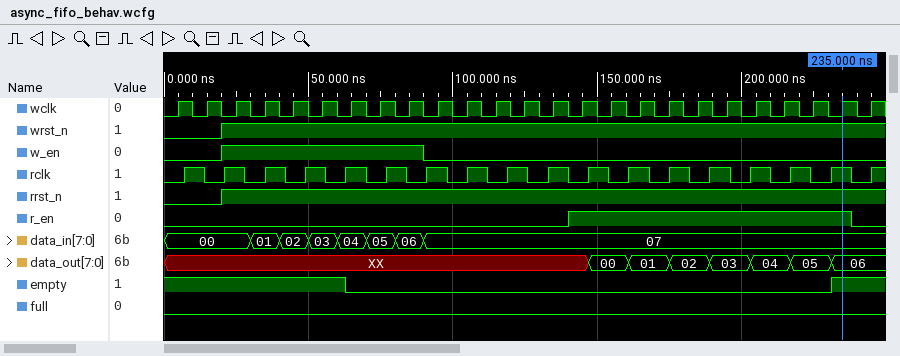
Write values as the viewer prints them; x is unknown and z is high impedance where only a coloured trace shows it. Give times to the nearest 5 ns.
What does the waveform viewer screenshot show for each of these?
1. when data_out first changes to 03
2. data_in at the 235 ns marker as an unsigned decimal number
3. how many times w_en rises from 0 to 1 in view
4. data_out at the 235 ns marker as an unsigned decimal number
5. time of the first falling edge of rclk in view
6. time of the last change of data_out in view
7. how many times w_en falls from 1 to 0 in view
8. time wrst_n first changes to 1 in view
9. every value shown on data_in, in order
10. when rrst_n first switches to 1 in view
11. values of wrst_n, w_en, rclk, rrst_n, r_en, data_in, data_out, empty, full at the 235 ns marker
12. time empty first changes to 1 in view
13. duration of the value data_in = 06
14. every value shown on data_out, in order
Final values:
190 ns
7
1
6
15 ns
230 ns
1
20 ns
00, 01, 02, 03, 04, 05, 06, 07
20 ns
wrst_n=1, w_en=0, rclk=1, rrst_n=1, r_en=1, data_in=07, data_out=06, empty=1, full=0
230 ns
10 ns
XX, 00, 01, 02, 03, 04, 05, 06
